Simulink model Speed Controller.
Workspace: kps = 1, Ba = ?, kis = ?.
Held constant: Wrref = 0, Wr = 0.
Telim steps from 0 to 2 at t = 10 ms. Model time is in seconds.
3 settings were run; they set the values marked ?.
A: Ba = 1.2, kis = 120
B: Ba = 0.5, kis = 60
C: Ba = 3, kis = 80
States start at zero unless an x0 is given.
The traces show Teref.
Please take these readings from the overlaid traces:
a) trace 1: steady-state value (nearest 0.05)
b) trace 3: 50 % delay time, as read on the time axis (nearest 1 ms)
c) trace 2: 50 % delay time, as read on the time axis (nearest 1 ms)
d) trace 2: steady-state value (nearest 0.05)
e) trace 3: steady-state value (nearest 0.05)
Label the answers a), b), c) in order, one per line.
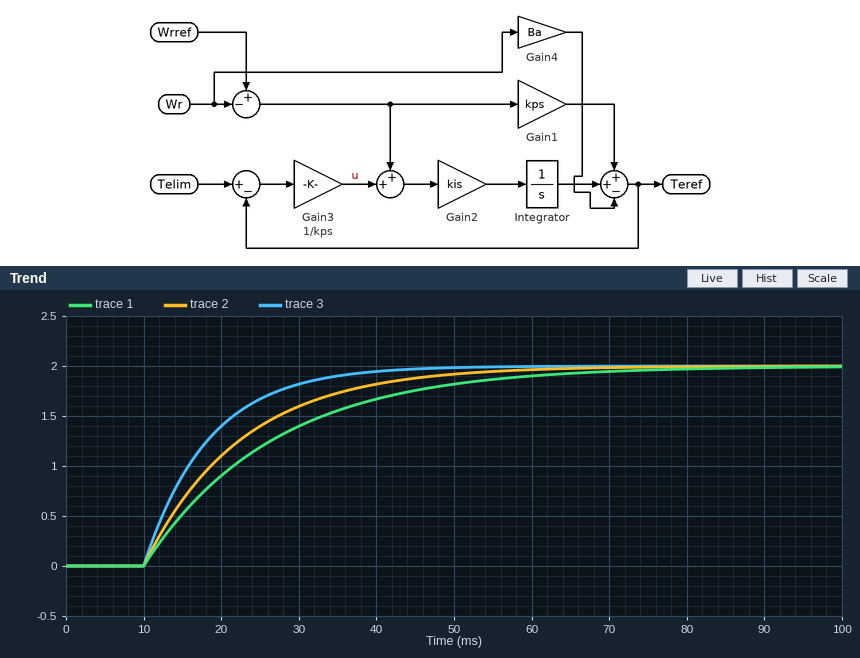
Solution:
a) 2.00
b) 16 ms
c) 19 ms
d) 2.00
e) 2.00
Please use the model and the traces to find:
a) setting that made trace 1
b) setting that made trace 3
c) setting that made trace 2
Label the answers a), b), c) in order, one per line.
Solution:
a) B
b) A
c) C
